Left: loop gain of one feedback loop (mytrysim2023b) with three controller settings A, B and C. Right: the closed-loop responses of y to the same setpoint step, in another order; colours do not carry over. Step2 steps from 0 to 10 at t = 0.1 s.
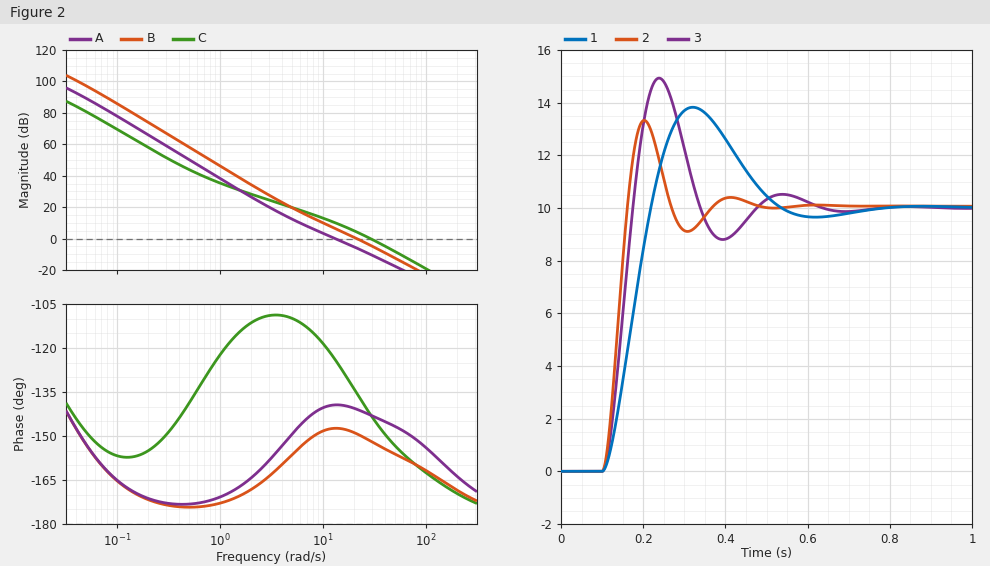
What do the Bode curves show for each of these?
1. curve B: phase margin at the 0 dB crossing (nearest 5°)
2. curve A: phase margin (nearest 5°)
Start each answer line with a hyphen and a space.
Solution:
- 30°
- 40°
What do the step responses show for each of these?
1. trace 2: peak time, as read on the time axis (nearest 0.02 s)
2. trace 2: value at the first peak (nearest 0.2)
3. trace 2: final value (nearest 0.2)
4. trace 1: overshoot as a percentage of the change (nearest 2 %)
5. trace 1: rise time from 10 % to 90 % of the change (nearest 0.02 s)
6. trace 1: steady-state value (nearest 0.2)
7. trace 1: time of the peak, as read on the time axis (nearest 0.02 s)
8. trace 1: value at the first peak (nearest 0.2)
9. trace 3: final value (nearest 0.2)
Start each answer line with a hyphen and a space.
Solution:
- 0.20 s
- 13.4
- 10.0
- 38 %
- 0.08 s
- 10.0
- 0.32 s
- 13.8
- 10.0
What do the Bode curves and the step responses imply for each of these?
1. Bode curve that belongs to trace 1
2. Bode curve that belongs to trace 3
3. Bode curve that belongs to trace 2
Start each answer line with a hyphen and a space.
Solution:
- A
- B
- C
